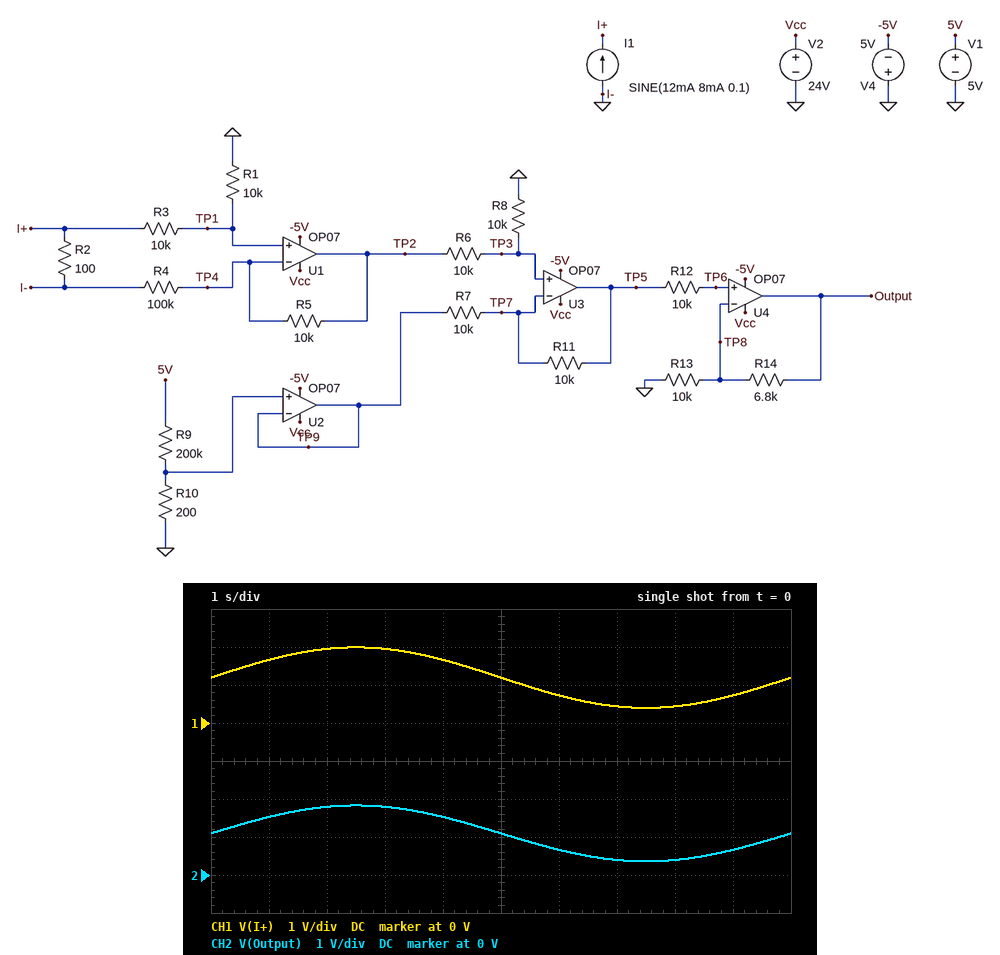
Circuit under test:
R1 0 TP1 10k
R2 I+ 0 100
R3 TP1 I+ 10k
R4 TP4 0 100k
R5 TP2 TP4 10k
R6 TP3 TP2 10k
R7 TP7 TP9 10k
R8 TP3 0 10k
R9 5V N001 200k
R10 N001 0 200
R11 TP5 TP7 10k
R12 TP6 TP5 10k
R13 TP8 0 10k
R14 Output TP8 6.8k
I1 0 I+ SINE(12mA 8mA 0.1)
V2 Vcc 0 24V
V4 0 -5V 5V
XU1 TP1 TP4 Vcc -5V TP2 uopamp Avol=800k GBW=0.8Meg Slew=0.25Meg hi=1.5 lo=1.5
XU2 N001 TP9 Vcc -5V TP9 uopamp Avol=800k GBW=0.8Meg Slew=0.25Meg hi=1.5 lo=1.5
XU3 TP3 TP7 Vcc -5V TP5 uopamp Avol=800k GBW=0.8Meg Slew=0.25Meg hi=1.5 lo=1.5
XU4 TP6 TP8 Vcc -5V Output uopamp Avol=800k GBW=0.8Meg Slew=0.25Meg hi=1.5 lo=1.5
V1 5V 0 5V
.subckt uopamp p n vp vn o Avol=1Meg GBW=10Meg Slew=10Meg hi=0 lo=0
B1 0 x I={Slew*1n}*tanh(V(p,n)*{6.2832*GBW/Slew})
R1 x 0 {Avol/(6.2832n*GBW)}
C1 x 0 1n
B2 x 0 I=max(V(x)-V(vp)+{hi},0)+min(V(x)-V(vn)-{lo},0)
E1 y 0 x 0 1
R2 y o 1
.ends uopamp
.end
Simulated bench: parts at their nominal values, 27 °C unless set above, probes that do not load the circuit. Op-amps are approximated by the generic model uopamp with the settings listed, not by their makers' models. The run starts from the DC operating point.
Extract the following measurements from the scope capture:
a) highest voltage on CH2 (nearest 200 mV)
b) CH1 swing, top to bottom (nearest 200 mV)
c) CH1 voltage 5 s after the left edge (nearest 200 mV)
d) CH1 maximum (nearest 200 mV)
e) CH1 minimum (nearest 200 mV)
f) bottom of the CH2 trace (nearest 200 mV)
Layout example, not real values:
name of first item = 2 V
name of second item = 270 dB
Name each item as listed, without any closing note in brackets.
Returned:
highest voltage on CH2 = 1.8 V
CH1 swing, top to bottom = 1.6 V
CH1 voltage 5 s after the left edge = 1.2 V
CH1 maximum = 2.0 V
CH1 minimum = 400 mV
bottom of the CH2 trace = 400 mV
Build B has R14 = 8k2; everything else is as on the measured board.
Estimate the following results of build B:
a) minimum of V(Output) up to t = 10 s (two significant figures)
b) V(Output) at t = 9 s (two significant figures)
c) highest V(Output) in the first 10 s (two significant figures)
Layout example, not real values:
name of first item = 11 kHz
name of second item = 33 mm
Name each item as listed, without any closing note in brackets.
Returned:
minimum of V(Output) up to t = 10 s = 390 mV
V(Output) at t = 9 s = 720 mV
highest V(Output) in the first 10 s = 2.0 V
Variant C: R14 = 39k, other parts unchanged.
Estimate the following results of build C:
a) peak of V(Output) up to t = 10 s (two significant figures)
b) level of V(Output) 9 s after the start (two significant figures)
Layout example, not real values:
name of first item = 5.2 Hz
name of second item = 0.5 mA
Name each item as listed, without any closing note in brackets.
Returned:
peak of V(Output) up to t = 10 s = 5.3 V
level of V(Output) 9 s after the start = 1.9 V
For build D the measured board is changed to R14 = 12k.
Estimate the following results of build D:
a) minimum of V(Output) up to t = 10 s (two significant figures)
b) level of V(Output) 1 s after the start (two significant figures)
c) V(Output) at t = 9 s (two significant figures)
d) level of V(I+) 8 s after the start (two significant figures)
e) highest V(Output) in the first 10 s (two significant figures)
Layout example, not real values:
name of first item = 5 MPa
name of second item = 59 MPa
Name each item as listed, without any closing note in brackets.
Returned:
minimum of V(Output) up to t = 10 s = 470 mV
level of V(Output) 1 s after the start = 2.0 V
V(Output) at t = 9 s = 870 mV
level of V(I+) 8 s after the start = 440 mV
highest V(Output) in the first 10 s = 2.4 V
